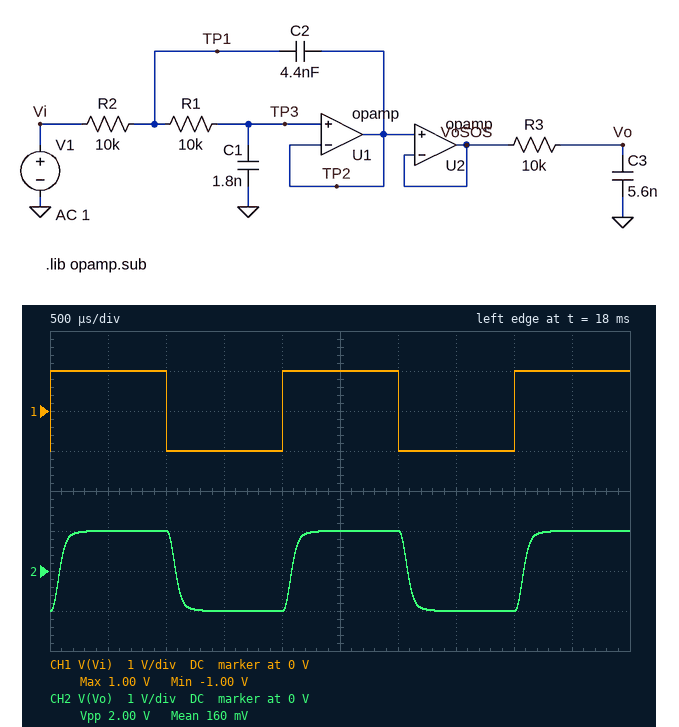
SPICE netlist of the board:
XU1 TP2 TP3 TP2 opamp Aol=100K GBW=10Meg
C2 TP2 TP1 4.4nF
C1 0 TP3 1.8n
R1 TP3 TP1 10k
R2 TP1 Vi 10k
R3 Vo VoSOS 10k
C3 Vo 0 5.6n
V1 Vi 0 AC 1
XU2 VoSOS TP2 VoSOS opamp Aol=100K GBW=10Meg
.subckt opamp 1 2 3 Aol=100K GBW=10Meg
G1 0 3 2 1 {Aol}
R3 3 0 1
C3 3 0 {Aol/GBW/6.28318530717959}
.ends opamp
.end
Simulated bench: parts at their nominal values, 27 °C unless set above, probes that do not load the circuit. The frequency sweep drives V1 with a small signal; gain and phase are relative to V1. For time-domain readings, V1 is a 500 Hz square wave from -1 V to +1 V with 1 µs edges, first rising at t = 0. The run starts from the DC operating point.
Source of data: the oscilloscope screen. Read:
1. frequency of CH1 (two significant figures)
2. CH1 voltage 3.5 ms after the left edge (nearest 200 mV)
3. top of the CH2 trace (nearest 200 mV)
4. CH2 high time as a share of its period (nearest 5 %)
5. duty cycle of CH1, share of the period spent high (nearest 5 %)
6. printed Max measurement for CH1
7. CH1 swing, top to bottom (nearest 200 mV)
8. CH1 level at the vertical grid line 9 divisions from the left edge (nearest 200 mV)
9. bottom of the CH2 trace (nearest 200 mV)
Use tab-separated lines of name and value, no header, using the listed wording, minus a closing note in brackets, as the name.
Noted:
frequency of CH1	500 Hz
CH1 voltage 3.5 ms after the left edge	-1.0 V
top of the CH2 trace	1.0 V
CH2 high time as a share of its period	50 %
duty cycle of CH1, share of the period spent high	50 %
printed Max measurement for CH1	1.00 V
CH1 swing, top to bottom	2.0 V
CH1 level at the vertical grid line 9 divisions from the left edge	1.0 V
bottom of the CH2 trace	-1.0 V
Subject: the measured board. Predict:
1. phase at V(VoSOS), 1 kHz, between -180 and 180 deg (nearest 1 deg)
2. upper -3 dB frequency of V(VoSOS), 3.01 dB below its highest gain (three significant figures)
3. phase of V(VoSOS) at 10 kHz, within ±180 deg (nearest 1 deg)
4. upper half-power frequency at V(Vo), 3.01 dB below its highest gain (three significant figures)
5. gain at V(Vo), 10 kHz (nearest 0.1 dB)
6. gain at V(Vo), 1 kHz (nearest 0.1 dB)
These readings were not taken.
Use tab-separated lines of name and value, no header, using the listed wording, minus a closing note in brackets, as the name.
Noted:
phase at V(VoSOS), 1 kHz, between -180 and 180 deg	-13 deg
upper -3 dB frequency of V(VoSOS), 3.01 dB below its highest gain	6.10 kHz
phase of V(VoSOS) at 10 kHz, within ±180 deg	-133 deg
upper half-power frequency at V(Vo), 3.01 dB below its highest gain	2.92 kHz
gain at V(Vo), 10 kHz	-21.1 dB
gain at V(Vo), 1 kHz	-0.5 dB
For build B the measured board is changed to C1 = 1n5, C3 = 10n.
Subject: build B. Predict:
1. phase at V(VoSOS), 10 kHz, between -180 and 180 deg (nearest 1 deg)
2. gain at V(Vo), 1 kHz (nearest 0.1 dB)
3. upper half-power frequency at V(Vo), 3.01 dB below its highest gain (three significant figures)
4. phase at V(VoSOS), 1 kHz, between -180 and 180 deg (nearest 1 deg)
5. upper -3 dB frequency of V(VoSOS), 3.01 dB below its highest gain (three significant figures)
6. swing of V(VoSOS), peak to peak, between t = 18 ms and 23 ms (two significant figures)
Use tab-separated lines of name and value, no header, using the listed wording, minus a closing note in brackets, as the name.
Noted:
phase at V(VoSOS), 10 kHz, between -180 and 180 deg	-131 deg
gain at V(Vo), 1 kHz	-1.4 dB
upper half-power frequency at V(Vo), 3.01 dB below its highest gain	1.66 kHz
phase at V(VoSOS), 1 kHz, between -180 and 180 deg	-11 deg
upper -3 dB frequency of V(VoSOS), 3.01 dB below its highest gain	6.97 kHz
swing of V(VoSOS), peak to peak, between t = 18 ms and 23 ms	2.4 V
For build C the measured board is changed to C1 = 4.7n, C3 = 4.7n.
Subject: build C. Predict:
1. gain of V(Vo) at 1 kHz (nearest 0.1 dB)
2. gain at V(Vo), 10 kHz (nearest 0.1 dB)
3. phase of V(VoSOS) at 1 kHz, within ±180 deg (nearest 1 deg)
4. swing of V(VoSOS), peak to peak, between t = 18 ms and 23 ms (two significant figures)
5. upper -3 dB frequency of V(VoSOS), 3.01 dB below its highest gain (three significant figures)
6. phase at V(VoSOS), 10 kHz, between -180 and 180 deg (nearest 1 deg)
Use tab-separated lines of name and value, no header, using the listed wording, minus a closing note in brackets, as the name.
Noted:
gain of V(Vo) at 1 kHz	-1.1 dB
gain at V(Vo), 10 kHz	-29.2 dB
phase of V(VoSOS) at 1 kHz, within ±180 deg	-33 deg
swing of V(VoSOS), peak to peak, between t = 18 ms and 23 ms	2.0 V
upper -3 dB frequency of V(VoSOS), 3.01 dB below its highest gain	2.15 kHz
phase at V(VoSOS), 10 kHz, between -180 and 180 deg	-141 deg
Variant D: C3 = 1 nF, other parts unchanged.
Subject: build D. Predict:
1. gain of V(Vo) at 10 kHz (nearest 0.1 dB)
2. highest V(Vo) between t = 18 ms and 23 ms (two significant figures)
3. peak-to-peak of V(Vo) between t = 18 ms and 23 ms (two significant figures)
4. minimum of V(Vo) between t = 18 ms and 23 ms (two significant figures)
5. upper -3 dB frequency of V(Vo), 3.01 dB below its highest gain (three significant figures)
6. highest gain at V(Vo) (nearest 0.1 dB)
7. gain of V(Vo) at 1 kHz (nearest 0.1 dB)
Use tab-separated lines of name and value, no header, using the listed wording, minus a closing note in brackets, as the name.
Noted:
gain of V(Vo) at 10 kHz	-11.3 dB
highest V(Vo) between t = 18 ms and 23 ms	1.1 V
peak-to-peak of V(Vo) between t = 18 ms and 23 ms	2.3 V
minimum of V(Vo) between t = 18 ms and 23 ms	-1.1 V
upper -3 dB frequency of V(Vo), 3.01 dB below its highest gain	5.82 kHz
highest gain at V(Vo)	0.1 dB
gain of V(Vo) at 1 kHz	0 dB
